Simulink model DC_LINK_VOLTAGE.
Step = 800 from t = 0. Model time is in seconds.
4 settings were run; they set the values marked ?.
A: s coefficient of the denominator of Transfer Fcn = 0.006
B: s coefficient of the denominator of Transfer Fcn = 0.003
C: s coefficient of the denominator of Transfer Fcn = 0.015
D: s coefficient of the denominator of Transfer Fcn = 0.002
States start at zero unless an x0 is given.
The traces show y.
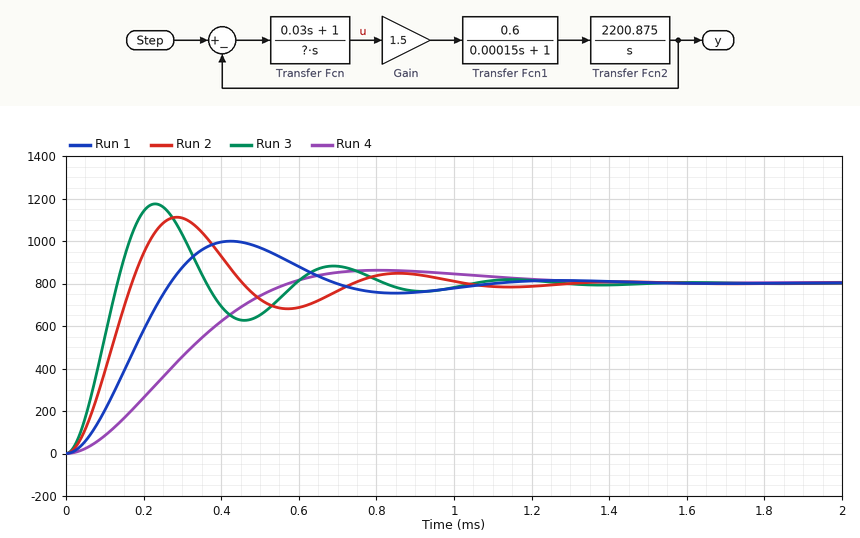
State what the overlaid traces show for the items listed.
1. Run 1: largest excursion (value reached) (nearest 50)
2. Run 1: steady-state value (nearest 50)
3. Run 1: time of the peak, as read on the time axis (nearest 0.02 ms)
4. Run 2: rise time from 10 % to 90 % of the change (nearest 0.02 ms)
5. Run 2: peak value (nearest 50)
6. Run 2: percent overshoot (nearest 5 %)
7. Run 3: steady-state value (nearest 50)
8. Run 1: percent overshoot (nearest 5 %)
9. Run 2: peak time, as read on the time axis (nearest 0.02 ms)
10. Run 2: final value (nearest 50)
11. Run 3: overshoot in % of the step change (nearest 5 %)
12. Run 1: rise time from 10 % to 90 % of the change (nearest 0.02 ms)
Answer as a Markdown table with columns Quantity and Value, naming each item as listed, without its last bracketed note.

| Quantity | Value |
|---|---|
| Run 1: largest excursion (value reached) | 1000 |
| Run 1: steady-state value | 800 |
| Run 1: time of the peak, as read on the time axis | 0.42 ms |
| Run 2: rise time from 10 % to 90 % of the change | 0.12 ms |
| Run 2: peak value | 1100 |
| Run 2: percent overshoot | 40 % |
| Run 3: steady-state value | 800 |
| Run 1: percent overshoot | 25 % |
| Run 2: peak time, as read on the time axis | 0.28 ms |
| Run 2: final value | 800 |
| Run 3: overshoot in % of the step change | 45 % |
| Run 1: rise time from 10 % to 90 % of the change | 0.18 ms |
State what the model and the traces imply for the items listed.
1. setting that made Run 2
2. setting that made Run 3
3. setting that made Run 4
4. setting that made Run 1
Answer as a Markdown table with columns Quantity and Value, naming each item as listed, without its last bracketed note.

| Quantity | Value |
|---|---|
| setting that made Run 2 | B |
| setting that made Run 3 | D |
| setting that made Run 4 | C |
| setting that made Run 1 | A |
